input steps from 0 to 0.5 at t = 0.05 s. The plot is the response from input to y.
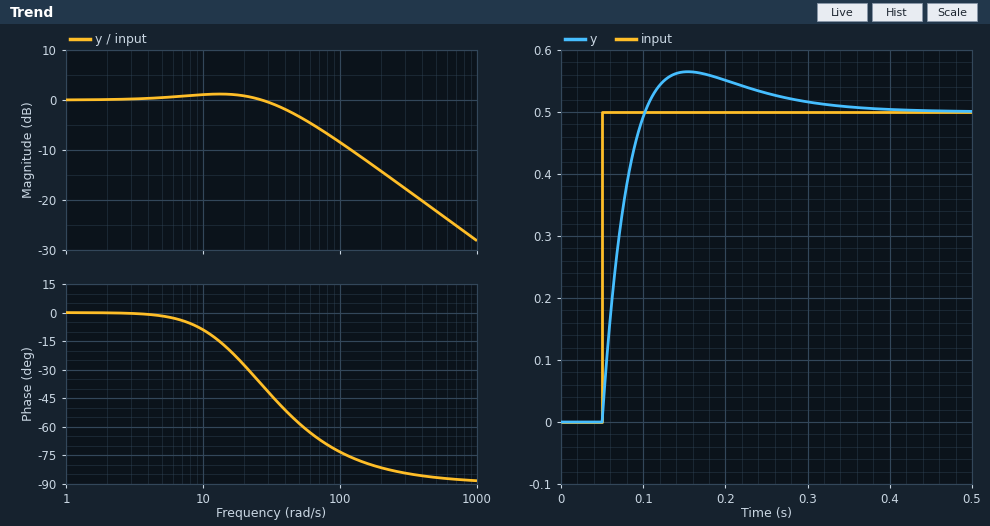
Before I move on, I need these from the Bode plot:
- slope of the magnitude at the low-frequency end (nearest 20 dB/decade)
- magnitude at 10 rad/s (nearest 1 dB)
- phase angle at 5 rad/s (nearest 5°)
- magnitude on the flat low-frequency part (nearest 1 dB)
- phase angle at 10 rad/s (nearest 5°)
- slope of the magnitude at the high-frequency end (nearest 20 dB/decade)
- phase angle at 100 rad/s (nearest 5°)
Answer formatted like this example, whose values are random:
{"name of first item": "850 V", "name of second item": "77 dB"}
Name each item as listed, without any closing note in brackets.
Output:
{"slope of the magnitude at the low-frequency end": "0 dB/decade", "magnitude at 10 rad/s": "1 dB", "phase angle at 5 rad/s": "0°", "magnitude on the flat low-frequency part": "0 dB", "phase angle at 10 rad/s": "-10°", "slope of the magnitude at the high-frequency end": "-20 dB/decade", "phase angle at 100 rad/s": "-75°"}
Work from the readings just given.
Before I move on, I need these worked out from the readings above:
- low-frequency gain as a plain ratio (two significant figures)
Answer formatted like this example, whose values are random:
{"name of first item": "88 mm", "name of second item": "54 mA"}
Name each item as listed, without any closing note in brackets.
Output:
{"low-frequency gain as a plain ratio": "1.0"}
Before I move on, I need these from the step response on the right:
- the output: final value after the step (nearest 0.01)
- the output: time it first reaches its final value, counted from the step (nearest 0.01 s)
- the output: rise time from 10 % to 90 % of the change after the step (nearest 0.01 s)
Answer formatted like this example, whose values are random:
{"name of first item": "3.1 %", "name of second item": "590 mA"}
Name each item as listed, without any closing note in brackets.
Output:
{"the output: final value after the step": "0.50", "the output: time it first reaches its final value, counted from the step": "0.05 s", "the output: rise time from 10 % to 90 % of the change after the step": "0.04 s"}
